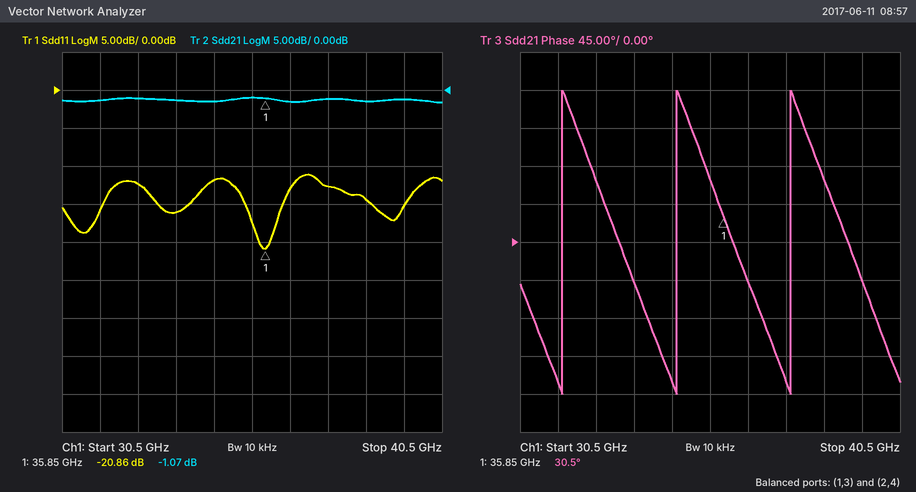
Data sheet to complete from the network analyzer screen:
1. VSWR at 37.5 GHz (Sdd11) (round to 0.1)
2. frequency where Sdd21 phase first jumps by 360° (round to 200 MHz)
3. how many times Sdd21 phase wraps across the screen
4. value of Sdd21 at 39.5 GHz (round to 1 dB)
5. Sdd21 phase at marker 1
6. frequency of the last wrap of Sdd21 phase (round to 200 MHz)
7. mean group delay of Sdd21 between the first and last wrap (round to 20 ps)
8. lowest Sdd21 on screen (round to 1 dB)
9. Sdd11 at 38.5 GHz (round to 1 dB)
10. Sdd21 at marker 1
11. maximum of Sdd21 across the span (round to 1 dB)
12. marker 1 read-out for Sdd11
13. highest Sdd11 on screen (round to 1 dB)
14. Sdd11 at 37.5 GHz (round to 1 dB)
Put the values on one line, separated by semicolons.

1.6; 31.6 GHz; 3; -1 dB; 30.5°; 37.6 GHz; 340 ps; -2 dB; -14 dB; -1.07 dB; -1 dB; -20.86 dB; -11 dB; -13 dB
